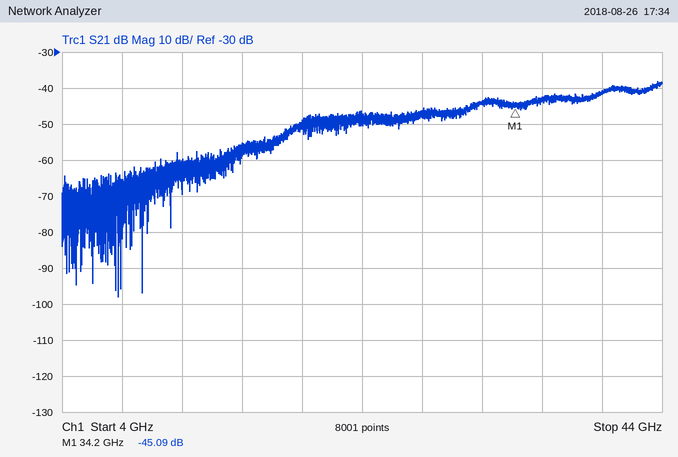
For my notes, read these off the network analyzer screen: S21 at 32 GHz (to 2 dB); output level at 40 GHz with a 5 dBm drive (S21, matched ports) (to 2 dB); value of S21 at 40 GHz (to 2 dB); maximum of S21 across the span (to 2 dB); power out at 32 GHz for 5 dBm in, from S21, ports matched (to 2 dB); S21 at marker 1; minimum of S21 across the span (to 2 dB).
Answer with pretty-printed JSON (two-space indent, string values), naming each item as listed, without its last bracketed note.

{
  "S21 at 32 GHz": "-44 dB",
  "output level at 40 GHz with a 5 dBm drive (S21, matched ports)": "-36 dBm",
  "value of S21 at 40 GHz": "-42 dB",
  "maximum of S21 across the span": "-38 dB",
  "power out at 32 GHz for 5 dBm in, from S21, ports matched": "-40 dBm",
  "S21 at marker 1": "-45.09 dB",
  "minimum of S21 across the span": "-98 dB"
}
